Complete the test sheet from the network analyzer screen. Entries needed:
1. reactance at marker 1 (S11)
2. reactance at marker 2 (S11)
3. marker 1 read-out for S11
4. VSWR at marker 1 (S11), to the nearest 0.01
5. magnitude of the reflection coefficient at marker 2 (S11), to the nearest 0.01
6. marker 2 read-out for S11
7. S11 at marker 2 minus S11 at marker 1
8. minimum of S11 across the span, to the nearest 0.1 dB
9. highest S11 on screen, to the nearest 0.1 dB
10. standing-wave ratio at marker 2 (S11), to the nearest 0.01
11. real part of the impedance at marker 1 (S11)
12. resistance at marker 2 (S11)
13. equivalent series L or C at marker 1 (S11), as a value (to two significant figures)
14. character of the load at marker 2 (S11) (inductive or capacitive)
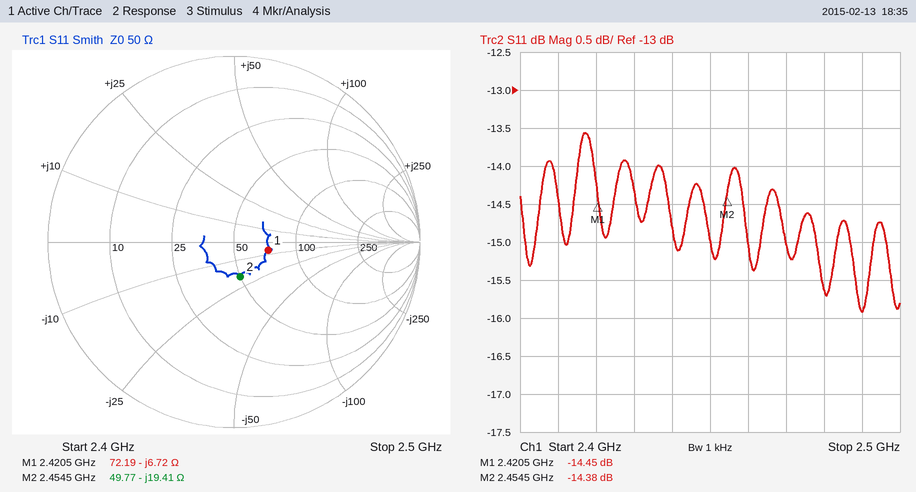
-6.72 Ω
-19.41 Ω
-14.45 dB
1.47
0.19
-14.38 dB
0.07 dB
-15.9 dB
-13.6 dB
1.47
72.19 Ω
49.77 Ω
9.8 pF
capacitive
